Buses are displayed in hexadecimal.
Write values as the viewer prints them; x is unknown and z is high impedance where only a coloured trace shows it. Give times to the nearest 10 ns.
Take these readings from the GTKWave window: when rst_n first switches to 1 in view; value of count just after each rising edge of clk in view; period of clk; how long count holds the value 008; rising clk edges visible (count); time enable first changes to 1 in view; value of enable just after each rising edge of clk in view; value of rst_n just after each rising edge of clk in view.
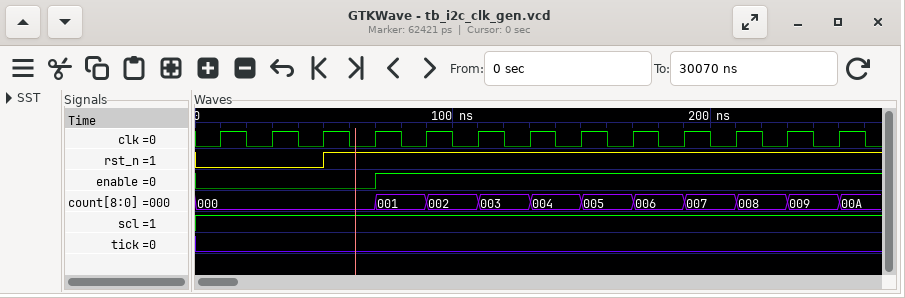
50 ns
000, 000, 000, 001, 002, 003, 004, 005, 006, 007, 008, 009, 00A
20 ns
20 ns
13
70 ns
0 0 0 1 1 1 1 1 1 1 1 1 1
0 0 1 1 1 1 1 1 1 1 1 1 1
